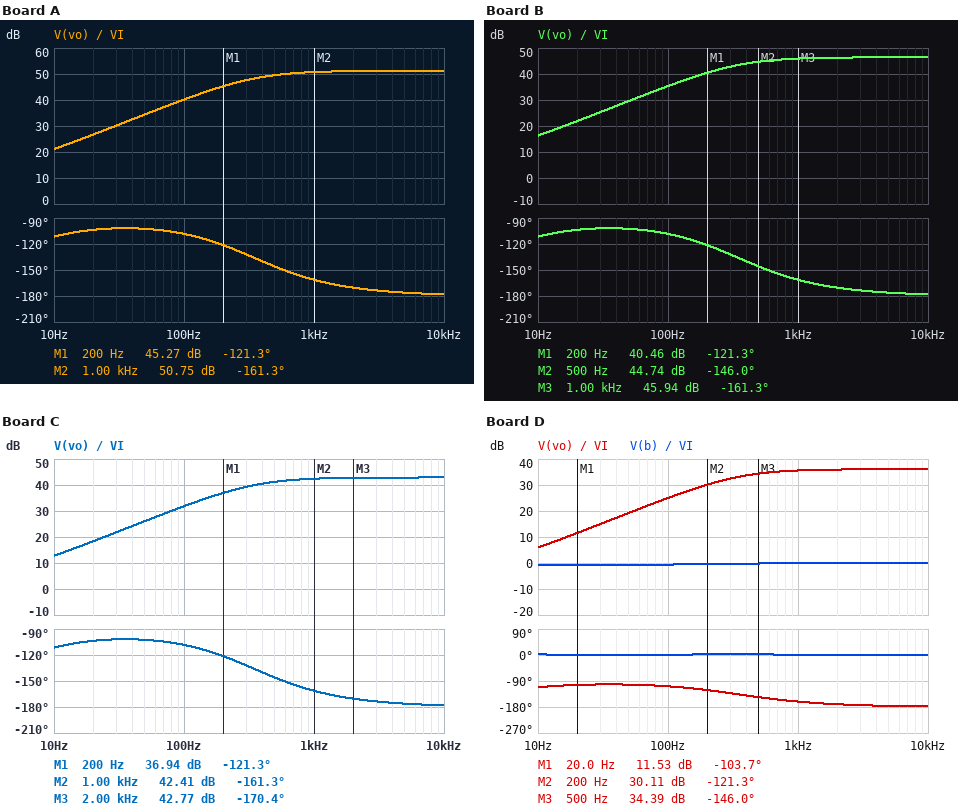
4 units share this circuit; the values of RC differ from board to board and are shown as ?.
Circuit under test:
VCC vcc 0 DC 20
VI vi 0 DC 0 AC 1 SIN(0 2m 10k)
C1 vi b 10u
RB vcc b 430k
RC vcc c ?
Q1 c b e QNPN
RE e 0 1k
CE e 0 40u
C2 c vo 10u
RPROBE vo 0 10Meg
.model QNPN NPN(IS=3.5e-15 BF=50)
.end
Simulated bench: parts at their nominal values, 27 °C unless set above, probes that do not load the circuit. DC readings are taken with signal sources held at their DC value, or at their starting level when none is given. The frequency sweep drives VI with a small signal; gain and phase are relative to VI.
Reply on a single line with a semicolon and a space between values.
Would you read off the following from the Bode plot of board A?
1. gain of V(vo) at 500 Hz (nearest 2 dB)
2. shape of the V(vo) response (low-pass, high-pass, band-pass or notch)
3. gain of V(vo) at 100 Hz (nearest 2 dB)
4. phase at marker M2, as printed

50 dB; high-pass; 40 dB; -161.3 deg
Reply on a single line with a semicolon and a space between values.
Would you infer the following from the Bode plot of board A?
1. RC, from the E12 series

4.7 kΩ
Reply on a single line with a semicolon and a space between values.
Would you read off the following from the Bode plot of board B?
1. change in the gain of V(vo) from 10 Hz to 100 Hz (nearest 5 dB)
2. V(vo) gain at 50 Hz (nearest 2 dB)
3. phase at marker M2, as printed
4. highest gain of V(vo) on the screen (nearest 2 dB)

20 dB; 30 dB; -146.0 deg; 46 dB
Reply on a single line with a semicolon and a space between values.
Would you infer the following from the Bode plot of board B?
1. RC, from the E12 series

2.7 kΩ
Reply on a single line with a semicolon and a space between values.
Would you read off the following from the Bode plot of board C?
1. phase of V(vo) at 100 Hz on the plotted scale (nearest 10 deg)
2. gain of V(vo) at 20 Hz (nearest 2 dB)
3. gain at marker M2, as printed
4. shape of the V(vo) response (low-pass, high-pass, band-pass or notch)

-110 deg; 18 dB; 42.41 dB; high-pass
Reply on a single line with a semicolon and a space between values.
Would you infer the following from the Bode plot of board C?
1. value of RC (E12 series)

1.8 kΩ
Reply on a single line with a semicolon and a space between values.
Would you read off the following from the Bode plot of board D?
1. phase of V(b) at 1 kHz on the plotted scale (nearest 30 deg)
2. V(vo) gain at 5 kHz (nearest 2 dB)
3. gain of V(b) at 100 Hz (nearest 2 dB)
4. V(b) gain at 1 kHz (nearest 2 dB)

0 deg; 36 dB; 0 dB; 0 dB
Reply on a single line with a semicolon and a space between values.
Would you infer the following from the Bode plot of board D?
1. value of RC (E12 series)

820 Ω
